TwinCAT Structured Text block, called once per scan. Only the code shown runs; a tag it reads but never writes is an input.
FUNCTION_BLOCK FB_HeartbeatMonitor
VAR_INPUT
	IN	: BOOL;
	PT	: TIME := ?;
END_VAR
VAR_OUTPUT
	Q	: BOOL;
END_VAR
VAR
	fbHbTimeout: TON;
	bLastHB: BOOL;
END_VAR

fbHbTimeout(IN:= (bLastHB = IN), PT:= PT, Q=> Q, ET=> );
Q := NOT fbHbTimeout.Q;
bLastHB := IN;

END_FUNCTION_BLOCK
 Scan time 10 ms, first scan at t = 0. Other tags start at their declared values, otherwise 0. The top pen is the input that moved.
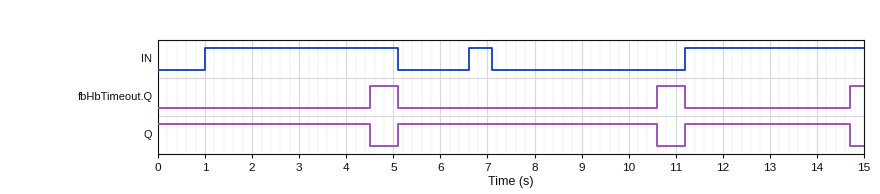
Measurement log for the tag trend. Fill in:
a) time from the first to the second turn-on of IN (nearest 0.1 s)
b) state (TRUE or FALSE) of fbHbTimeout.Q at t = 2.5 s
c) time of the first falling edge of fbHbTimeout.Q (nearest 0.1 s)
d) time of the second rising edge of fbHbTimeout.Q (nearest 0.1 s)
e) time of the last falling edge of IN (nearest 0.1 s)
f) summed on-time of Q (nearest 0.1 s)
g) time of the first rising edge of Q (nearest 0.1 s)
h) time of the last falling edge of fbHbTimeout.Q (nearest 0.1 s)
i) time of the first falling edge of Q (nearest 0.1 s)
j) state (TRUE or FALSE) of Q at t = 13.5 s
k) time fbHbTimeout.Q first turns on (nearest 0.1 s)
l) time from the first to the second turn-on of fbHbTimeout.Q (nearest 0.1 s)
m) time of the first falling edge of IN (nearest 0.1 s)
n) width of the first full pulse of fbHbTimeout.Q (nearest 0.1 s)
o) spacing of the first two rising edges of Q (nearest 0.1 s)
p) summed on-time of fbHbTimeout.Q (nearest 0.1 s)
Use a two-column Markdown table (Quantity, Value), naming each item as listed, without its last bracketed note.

| Quantity | Value |
|---|---|
| time from the first to the second turn-on of IN | 5.6 s |
| state (TRUE or FALSE) of fbHbTimeout.Q at t = 2.5 s | FALSE |
| time of the first falling edge of fbHbTimeout.Q | 5.1 s |
| time of the second rising edge of fbHbTimeout.Q | 10.6 s |
| time of the last falling edge of IN | 7.1 s |
| summed on-time of Q | 13.5 s |
| time of the first rising edge of Q | 5.1 s |
| time of the last falling edge of fbHbTimeout.Q | 11.2 s |
| time of the first falling edge of Q | 4.5 s |
| state (TRUE or FALSE) of Q at t = 13.5 s | TRUE |
| time fbHbTimeout.Q first turns on | 4.5 s |
| time from the first to the second turn-on of fbHbTimeout.Q | 6.1 s |
| time of the first falling edge of IN | 5.1 s |
| width of the first full pulse of fbHbTimeout.Q | 0.6 s |
| spacing of the first two rising edges of Q | 6.1 s |
| summed on-time of fbHbTimeout.Q | 1.5 s |
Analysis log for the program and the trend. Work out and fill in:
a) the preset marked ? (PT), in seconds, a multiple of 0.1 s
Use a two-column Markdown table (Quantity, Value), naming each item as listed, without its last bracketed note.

| Quantity | Value |
|---|---|
| the preset marked ? (PT), in seconds, a multiple of 0.1 s | 3.5 s |
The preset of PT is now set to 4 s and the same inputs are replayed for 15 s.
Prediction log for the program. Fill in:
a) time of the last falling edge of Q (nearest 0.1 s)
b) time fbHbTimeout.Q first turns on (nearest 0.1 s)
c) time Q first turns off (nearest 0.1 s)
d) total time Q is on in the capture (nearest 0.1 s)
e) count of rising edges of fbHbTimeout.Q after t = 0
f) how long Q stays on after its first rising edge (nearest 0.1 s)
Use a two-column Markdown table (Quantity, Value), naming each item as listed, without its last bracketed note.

| Quantity | Value |
|---|---|
| time of the last falling edge of Q | 11.1 s |
| time fbHbTimeout.Q first turns on | 5.0 s |
| time Q first turns off | 5.0 s |
| total time Q is on in the capture | 14.8 s |
| count of rising edges of fbHbTimeout.Q after t = 0 | 2 |
| how long Q stays on after its first rising edge | 6.0 s |
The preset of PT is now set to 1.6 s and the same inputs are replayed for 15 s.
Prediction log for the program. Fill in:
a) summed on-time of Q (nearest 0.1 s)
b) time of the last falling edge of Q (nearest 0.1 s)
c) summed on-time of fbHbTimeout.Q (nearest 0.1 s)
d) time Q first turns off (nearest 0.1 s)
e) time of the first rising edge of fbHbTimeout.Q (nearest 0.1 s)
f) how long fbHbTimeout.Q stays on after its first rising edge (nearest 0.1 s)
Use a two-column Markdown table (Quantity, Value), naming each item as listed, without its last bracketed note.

| Quantity | Value |
|---|---|
| summed on-time of Q | 7.8 s |
| time of the last falling edge of Q | 12.8 s |
| summed on-time of fbHbTimeout.Q | 7.2 s |
| time Q first turns off | 2.6 s |
| time of the first rising edge of fbHbTimeout.Q | 2.6 s |
| how long fbHbTimeout.Q stays on after its first rising edge | 2.5 s |
